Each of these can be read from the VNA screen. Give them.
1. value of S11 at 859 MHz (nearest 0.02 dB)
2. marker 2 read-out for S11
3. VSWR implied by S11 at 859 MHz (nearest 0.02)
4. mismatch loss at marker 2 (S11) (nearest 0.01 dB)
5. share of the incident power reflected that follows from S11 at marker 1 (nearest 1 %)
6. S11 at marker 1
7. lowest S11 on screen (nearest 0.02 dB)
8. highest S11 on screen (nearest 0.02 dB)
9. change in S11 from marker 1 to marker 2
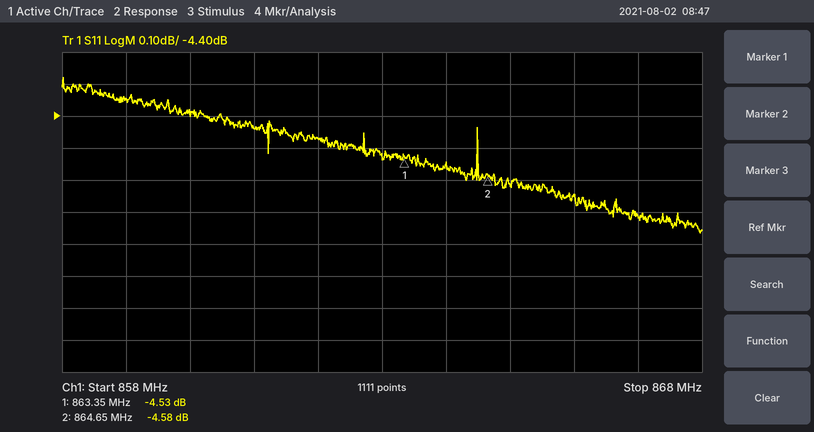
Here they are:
-4.34 dB
-4.58 dB
4.08
1.86 dB
35 %
-4.53 dB
-4.76 dB
-4.28 dB
-0.05 dB
